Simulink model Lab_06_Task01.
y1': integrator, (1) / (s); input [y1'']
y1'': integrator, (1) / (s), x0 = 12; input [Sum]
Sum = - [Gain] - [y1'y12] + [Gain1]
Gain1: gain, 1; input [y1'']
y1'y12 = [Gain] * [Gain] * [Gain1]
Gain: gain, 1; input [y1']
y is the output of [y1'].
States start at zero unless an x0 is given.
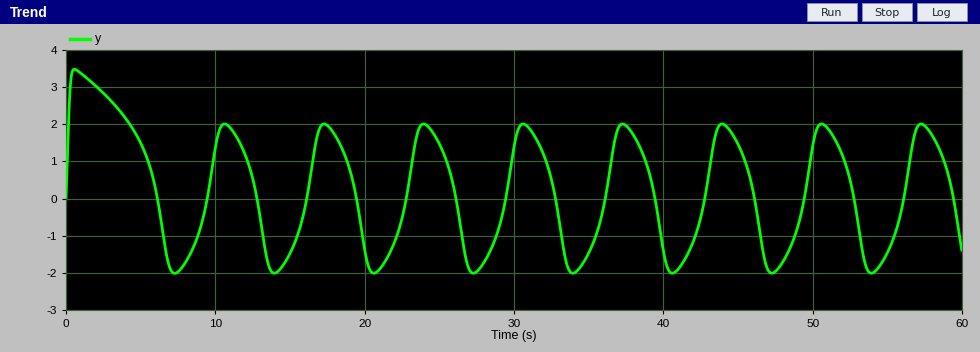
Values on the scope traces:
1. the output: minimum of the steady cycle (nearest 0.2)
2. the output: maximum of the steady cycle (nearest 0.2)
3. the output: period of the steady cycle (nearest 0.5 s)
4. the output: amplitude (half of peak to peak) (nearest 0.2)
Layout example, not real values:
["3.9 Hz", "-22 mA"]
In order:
["-2.0", "2.0", "6.5 s", "2.0"]
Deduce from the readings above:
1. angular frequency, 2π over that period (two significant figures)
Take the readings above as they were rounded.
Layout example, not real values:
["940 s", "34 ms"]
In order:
["0.97 rad/s"]
